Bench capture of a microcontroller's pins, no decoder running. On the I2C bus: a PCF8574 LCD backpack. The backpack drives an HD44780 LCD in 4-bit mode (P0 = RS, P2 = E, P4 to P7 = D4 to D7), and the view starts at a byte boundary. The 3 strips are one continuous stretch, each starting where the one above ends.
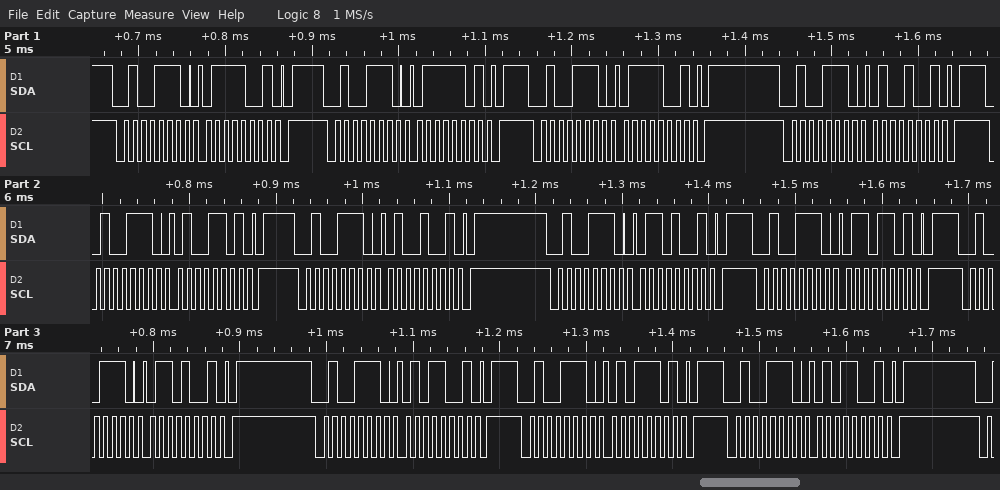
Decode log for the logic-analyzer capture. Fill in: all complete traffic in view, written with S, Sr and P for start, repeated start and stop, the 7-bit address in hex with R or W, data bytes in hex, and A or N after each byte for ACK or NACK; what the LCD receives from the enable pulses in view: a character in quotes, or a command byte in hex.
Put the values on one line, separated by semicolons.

S 27W A 79 A P S 27W A 7D A P S 27W A 79 A P S 27W A 49 A P S 27W A 4D A P S 27W A 49 A P S 27W A 69 A P S 27W A 6D A P S 27W A 69 A P S 27W A 59 A P S 27W A 5D A P S 27W A 59 A P; 't' 'e'
